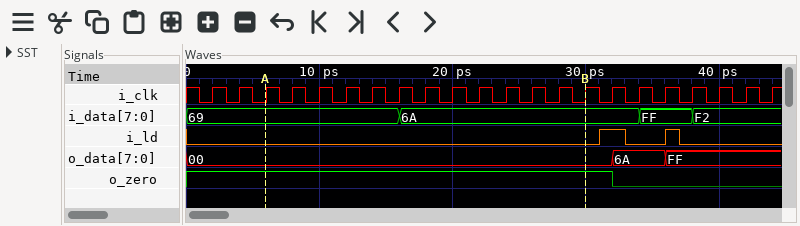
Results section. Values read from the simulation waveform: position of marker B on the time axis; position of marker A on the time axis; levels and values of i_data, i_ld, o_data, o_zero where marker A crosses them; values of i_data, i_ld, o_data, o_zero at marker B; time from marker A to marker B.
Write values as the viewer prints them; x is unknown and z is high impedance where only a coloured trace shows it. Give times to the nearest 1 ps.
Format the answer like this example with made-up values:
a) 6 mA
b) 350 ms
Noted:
a) 30 ps
b) 6 ps
c) i_data=69, i_ld=0, o_data=00, o_zero=1
d) i_data=6A, i_ld=0, o_data=00, o_zero=1
e) 24 ps
